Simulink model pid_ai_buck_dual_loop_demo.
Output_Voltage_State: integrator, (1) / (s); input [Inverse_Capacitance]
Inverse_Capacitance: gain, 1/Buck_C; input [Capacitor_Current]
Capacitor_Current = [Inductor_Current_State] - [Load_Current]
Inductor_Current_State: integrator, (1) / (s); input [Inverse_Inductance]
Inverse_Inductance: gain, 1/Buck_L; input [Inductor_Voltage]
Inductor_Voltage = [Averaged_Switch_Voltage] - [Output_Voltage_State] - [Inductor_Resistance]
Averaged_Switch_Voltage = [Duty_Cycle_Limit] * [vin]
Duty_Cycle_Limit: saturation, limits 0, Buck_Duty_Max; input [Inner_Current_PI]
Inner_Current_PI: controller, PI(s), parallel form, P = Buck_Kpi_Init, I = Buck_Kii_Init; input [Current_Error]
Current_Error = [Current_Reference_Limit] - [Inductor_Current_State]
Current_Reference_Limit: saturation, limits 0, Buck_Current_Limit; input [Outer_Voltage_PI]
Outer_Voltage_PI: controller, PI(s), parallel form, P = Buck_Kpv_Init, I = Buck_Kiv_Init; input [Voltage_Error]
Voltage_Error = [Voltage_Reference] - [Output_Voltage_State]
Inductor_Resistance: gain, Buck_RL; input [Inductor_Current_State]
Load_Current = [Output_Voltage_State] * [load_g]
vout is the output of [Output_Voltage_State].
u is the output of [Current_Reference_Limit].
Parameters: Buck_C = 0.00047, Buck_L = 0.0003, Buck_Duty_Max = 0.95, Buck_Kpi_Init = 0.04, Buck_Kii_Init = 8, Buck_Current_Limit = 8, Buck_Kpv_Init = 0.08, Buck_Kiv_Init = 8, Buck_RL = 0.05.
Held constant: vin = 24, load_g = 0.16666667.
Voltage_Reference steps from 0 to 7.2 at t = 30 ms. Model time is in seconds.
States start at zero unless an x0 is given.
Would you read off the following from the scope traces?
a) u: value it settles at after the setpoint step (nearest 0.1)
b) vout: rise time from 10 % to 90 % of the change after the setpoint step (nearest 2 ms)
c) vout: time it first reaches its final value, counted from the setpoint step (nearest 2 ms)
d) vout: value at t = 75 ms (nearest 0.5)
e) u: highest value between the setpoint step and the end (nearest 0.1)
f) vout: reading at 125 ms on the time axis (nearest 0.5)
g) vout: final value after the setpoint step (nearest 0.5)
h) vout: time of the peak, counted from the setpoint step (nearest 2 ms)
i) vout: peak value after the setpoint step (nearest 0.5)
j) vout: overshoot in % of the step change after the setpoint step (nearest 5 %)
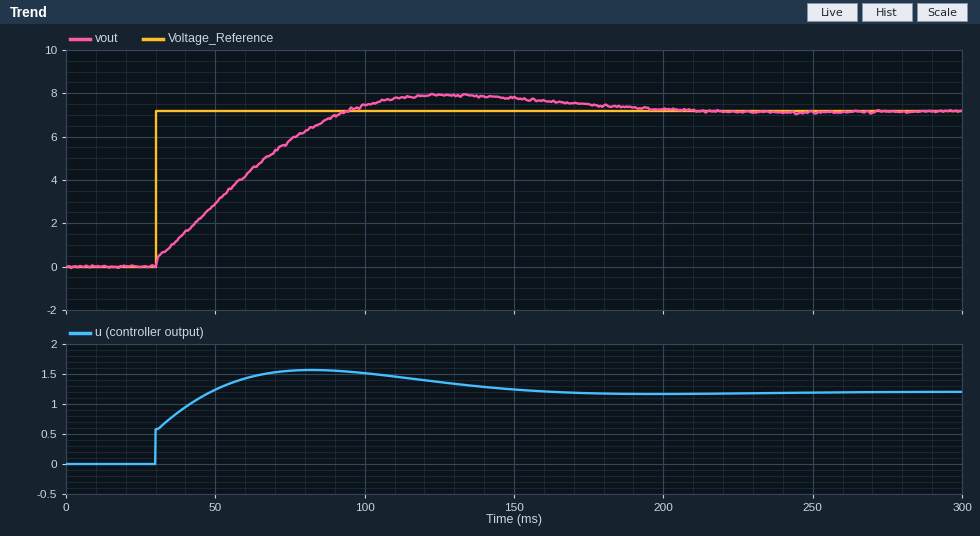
1.2
50 ms
64 ms
6.0
1.6
8.0
7.0
98 ms
8.0
10 %
